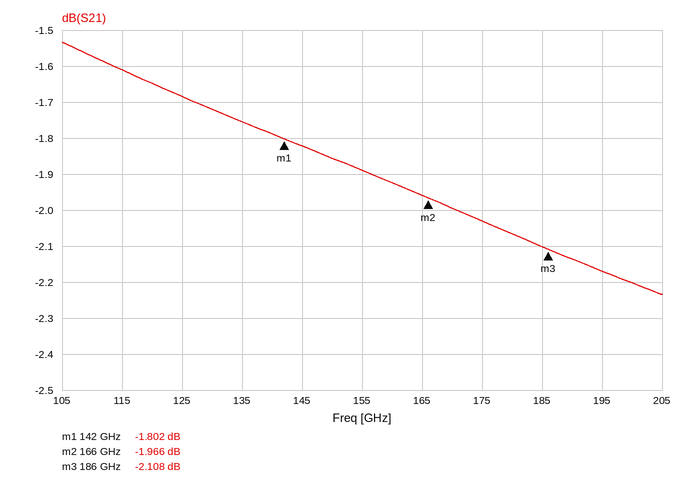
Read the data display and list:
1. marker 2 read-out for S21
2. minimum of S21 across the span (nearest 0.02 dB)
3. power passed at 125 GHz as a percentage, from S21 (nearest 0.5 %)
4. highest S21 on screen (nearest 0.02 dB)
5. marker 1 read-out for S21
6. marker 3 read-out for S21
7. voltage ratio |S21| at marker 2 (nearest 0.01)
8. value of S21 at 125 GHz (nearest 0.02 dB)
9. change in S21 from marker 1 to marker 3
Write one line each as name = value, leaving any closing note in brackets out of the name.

marker 2 read-out for S21 = -1.966 dB
minimum of S21 across the span = -2.24 dB
power passed at 125 GHz as a percentage, from S21 = 68.0 %
highest S21 on screen = -1.54 dB
marker 1 read-out for S21 = -1.802 dB
marker 3 read-out for S21 = -2.108 dB
voltage ratio |S21| at marker 2 = 0.80
value of S21 at 125 GHz = -1.68 dB
change in S21 from marker 1 to marker 3 = -0.306 dB
